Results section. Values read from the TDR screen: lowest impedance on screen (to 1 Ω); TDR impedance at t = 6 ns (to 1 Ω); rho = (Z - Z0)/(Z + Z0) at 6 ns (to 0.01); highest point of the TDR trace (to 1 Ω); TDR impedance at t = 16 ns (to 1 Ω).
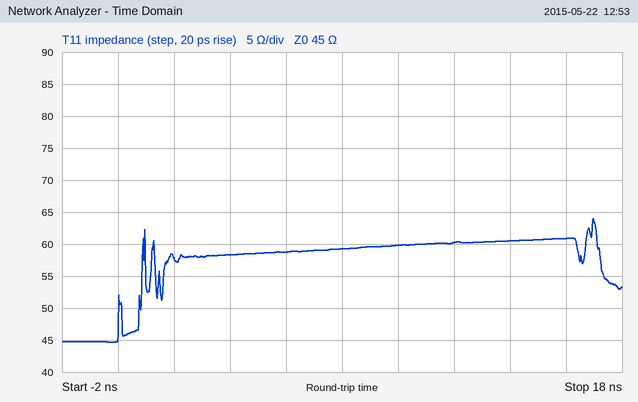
45 Ω
59 Ω
+0.13
64 Ω
61 Ω
